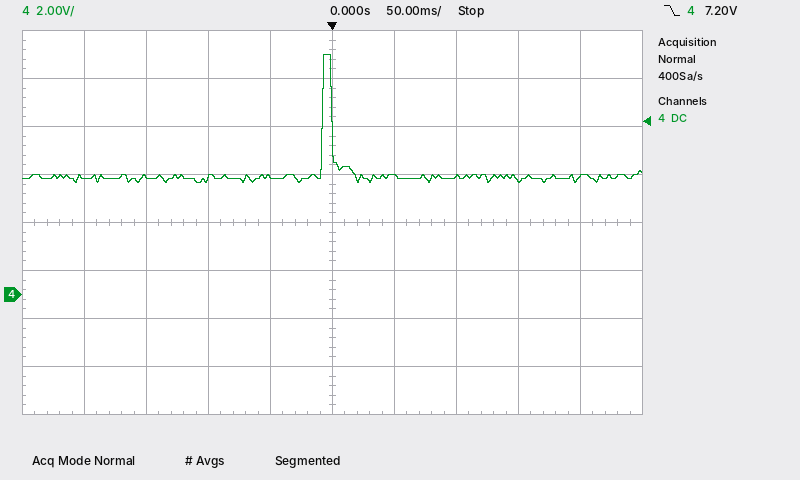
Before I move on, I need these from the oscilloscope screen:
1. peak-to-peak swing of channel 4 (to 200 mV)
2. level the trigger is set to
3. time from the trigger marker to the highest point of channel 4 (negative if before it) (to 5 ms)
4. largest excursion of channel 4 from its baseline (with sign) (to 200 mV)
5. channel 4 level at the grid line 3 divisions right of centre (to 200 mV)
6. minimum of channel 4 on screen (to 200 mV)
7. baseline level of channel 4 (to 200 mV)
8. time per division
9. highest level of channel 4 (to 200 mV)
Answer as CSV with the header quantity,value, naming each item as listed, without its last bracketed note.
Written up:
quantity,value
peak-to-peak swing of channel 4,5.4 V
level the trigger is set to,7.20 V
time from the trigger marker to the highest point of channel 4 (negative if before it),-5 ms
largest excursion of channel 4 from its baseline (with sign),+5.2 V
channel 4 level at the grid line 3 divisions right of centre,4.8 V
minimum of channel 4 on screen,4.6 V
baseline level of channel 4,4.8 V
time per division,50 ms
highest level of channel 4,10.0 V
